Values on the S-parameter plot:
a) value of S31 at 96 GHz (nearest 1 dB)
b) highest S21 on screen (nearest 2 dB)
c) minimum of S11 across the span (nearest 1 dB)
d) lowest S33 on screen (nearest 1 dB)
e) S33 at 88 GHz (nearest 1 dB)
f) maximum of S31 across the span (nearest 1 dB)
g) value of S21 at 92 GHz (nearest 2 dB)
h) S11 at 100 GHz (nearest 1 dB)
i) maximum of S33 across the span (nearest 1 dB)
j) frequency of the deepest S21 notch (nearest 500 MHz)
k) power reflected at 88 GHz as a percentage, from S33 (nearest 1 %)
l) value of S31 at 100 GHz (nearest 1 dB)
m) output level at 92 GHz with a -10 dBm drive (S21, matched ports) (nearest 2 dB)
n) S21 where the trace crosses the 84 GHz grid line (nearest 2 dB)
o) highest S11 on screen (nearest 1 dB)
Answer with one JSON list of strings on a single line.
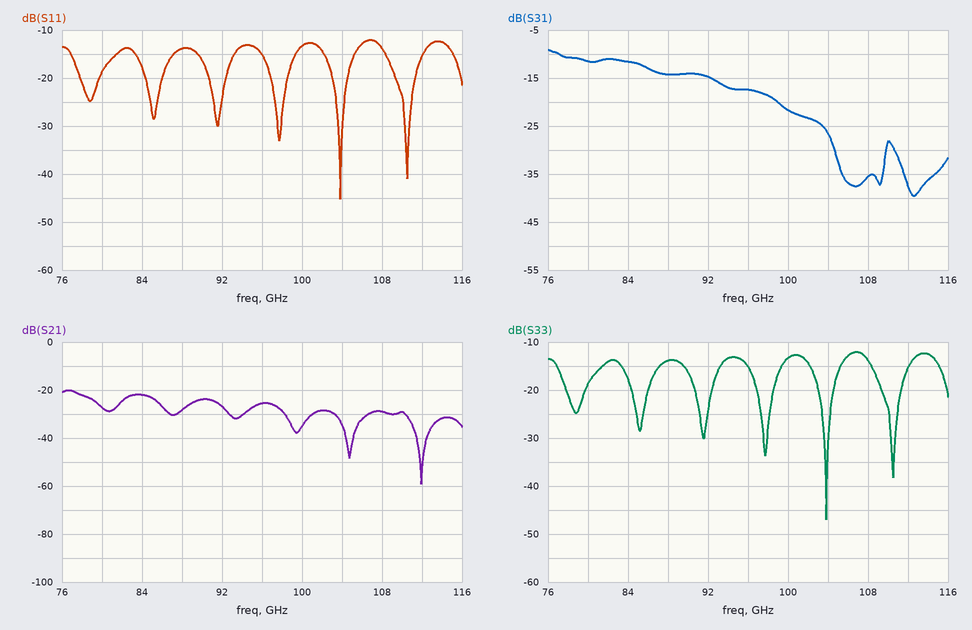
["-17 dB", "-20 dB", "-45 dB", "-47 dB", "-14 dB", "-9 dB", "-26 dB", "-13 dB", "-12 dB", "112.0 GHz", "4 %", "-22 dB", "-36 dBm", "-22 dB", "-12 dB"]
